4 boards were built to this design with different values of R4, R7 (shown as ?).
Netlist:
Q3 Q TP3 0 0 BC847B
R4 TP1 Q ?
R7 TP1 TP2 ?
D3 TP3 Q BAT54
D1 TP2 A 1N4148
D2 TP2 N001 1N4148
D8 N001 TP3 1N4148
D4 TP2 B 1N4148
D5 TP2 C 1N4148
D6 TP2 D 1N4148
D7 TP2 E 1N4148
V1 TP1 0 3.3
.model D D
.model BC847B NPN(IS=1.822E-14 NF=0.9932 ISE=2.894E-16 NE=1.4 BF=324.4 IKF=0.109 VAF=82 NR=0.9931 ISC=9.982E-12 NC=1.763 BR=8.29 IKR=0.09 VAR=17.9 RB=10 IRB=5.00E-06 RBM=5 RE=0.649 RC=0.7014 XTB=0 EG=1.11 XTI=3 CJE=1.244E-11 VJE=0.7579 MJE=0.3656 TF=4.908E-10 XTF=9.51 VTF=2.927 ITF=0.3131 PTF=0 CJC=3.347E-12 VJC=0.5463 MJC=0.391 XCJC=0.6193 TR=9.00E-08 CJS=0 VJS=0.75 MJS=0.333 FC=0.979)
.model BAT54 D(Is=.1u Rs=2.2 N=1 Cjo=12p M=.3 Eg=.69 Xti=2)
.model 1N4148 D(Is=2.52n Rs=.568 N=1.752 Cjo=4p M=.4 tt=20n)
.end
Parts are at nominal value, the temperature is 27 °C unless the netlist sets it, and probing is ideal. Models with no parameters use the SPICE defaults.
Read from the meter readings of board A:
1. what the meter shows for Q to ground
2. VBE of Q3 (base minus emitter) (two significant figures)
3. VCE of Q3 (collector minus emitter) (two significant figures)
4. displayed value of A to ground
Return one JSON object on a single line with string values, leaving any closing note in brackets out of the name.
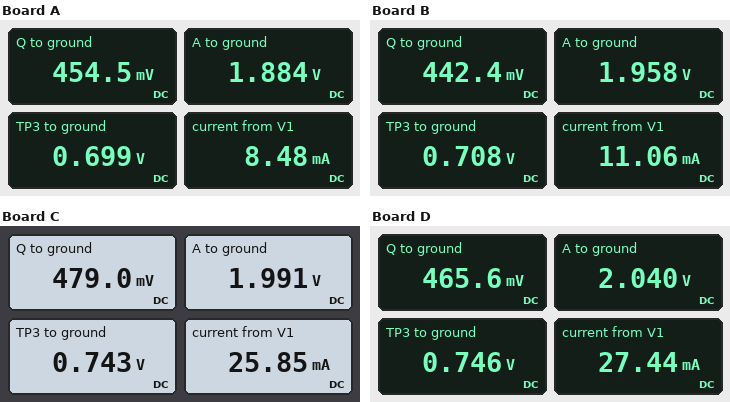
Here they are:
{"what the meter shows for Q to ground": "454.5 mV", "VBE of Q3 (base minus emitter)": "700 mV", "VCE of Q3 (collector minus emitter)": "450 mV", "displayed value of A to ground": "1.884 V"}
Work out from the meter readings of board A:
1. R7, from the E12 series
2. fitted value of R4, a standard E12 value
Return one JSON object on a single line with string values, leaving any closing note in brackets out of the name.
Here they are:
{"R7, from the E12 series": "1.2 kΩ", "fitted value of R4, a standard E12 value": "390 Ω"}
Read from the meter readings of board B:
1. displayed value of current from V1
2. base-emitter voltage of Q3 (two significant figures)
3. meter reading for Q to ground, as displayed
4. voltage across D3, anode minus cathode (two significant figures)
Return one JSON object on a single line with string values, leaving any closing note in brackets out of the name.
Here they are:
{"displayed value of current from V1": "11.06 mA", "base-emitter voltage of Q3": "710 mV", "meter reading for Q to ground, as displayed": "442.4 mV", "voltage across D3, anode minus cathode": "270 mV"}
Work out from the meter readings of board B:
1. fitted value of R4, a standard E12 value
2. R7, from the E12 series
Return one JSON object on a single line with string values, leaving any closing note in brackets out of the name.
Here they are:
{"fitted value of R4, a standard E12 value": "330 Ω", "R7, from the E12 series": "560 Ω"}
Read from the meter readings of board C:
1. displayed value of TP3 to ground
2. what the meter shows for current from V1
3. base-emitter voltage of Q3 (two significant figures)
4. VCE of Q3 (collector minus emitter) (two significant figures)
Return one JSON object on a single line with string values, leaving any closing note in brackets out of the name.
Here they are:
{"displayed value of TP3 to ground": "0.743 V", "what the meter shows for current from V1": "25.85 mA", "base-emitter voltage of Q3": "740 mV", "VCE of Q3 (collector minus emitter)": "480 mV"}
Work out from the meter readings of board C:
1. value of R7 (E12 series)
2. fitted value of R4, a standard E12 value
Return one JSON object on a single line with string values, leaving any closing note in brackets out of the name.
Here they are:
{"value of R7": "560 Ω", "fitted value of R4, a standard E12 value": "120 Ω"}
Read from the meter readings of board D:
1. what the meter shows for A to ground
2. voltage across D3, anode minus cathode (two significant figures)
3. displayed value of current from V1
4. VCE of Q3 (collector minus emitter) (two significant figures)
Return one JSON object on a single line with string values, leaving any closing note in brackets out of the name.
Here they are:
{"what the meter shows for A to ground": "2.040 V", "voltage across D3, anode minus cathode": "280 mV", "displayed value of current from V1": "27.44 mA", "VCE of Q3 (collector minus emitter)": "470 mV"}
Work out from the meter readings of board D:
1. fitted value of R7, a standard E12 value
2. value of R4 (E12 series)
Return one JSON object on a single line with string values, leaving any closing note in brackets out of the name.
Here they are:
{"fitted value of R7, a standard E12 value": "330 Ω", "value of R4": "120 Ω"}
